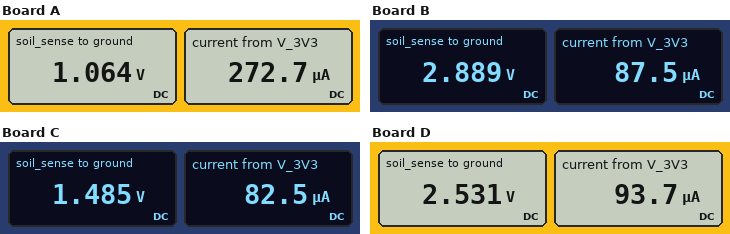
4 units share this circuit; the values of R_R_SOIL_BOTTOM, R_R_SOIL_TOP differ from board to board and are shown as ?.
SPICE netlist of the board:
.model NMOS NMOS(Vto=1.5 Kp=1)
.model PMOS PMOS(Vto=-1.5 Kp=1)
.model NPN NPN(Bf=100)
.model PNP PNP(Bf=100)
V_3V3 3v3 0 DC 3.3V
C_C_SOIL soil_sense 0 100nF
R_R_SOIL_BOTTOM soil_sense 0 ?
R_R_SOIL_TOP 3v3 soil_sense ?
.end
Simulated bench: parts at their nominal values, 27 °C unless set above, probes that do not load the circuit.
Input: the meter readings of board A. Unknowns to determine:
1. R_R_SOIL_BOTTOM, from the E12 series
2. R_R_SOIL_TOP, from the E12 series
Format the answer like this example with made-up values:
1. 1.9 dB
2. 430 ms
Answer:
1. 3.9 kΩ
2. 8.2 kΩ
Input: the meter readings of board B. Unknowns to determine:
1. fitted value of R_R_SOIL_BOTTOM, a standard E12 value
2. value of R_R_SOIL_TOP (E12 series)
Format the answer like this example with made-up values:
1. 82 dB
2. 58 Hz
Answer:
1. 33 kΩ
2. 4.7 kΩ
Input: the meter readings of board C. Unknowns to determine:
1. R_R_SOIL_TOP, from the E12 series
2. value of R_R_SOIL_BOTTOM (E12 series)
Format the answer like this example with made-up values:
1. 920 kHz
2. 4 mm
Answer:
1. 22 kΩ
2. 18 kΩ
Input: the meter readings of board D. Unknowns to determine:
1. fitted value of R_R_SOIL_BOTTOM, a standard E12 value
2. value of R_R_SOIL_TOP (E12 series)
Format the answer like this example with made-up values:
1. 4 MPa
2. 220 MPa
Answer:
1. 27 kΩ
2. 8.2 kΩ
